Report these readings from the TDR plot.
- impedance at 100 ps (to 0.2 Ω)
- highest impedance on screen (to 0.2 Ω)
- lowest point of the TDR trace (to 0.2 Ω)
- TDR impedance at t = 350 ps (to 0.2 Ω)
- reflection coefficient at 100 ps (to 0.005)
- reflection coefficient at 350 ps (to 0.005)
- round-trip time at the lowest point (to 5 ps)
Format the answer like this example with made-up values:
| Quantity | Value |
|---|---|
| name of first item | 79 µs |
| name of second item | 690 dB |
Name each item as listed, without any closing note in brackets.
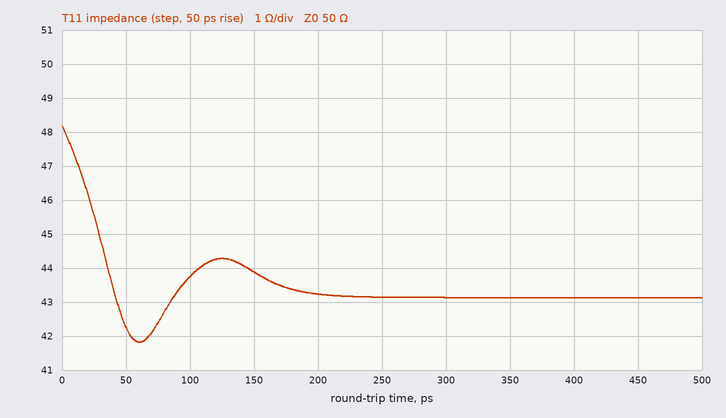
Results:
| Quantity | Value |
|---|---|
| impedance at 100 ps | 43.8 Ω |
| highest impedance on screen | 48.2 Ω |
| lowest point of the TDR trace | 41.8 Ω |
| TDR impedance at t = 350 ps | 43.2 Ω |
| reflection coefficient at 100 ps | -0.065 |
| reflection coefficient at 350 ps | -0.075 |
| round-trip time at the lowest point | 60 ps |
